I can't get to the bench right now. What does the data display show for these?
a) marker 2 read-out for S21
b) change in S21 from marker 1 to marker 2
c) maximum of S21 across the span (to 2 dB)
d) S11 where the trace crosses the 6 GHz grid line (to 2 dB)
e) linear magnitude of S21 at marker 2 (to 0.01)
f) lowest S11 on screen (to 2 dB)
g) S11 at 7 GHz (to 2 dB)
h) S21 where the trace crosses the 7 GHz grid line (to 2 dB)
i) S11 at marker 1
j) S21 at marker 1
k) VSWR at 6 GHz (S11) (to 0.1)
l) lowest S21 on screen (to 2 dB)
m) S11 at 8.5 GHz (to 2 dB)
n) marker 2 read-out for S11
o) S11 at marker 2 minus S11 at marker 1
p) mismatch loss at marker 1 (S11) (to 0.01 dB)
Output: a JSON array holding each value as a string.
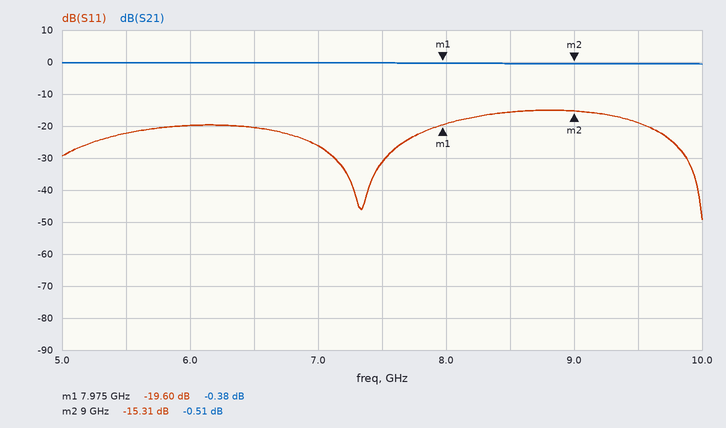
["-0.51 dB", "-0.13 dB", "0 dB", "-20 dB", "0.94", "-50 dB", "-26 dB", "0 dB", "-19.60 dB", "-0.38 dB", "1.2", "0 dB", "-16 dB", "-15.31 dB", "4.29 dB", "0.05 dB"]
